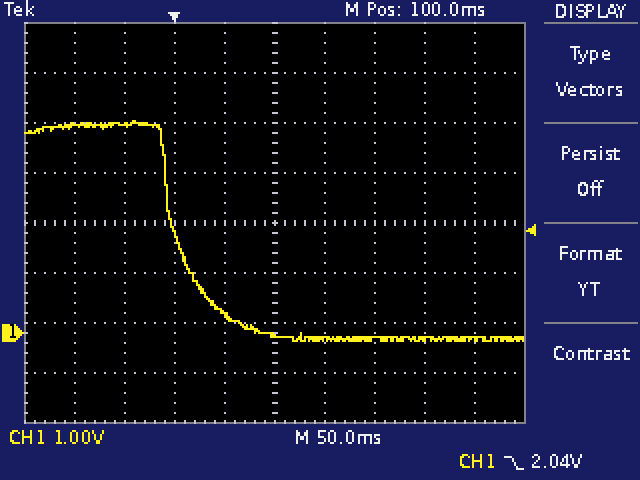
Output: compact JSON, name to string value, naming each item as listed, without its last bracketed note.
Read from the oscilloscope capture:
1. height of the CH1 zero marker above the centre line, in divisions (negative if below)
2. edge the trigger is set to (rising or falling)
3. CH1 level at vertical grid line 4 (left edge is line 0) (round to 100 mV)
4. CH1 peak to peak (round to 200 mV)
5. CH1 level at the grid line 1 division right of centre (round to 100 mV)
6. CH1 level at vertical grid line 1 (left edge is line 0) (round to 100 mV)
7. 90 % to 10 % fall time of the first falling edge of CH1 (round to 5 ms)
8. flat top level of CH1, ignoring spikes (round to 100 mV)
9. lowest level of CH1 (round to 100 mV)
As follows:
{"height of the CH1 zero marker above the centre line, in divisions": "-2.2 div", "edge the trigger is set to": "falling", "CH1 level at vertical grid line 4 (left edge is line 0)": "400 mV", "CH1 peak to peak": "4.4 V", "CH1 level at the grid line 1 division right of centre": "-100 mV", "CH1 level at vertical grid line 1 (left edge is line 0)": "4.2 V", "90 % to 10 % fall time of the first falling edge of CH1": "65 ms", "flat top level of CH1, ignoring spikes": "4.2 V", "lowest level of CH1": "-200 mV"}
